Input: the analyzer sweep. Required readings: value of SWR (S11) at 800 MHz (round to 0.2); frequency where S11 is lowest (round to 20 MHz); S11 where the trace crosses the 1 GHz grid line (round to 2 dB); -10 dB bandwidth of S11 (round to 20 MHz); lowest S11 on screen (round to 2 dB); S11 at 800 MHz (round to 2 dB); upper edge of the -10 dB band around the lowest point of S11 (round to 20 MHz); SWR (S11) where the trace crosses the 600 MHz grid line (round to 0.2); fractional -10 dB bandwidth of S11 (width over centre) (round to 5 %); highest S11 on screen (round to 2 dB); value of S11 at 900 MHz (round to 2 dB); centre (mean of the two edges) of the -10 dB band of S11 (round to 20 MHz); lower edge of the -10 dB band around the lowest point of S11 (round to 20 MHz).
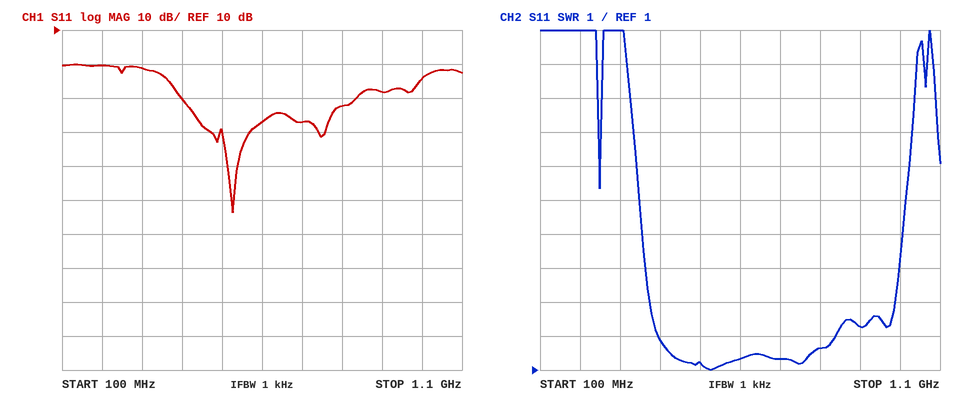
1.6
520 MHz
-4 dB
440 MHz
-44 dB
-12 dB
840 MHz
1.4
70 %
0 dB
-8 dB
620 MHz
400 MHz
